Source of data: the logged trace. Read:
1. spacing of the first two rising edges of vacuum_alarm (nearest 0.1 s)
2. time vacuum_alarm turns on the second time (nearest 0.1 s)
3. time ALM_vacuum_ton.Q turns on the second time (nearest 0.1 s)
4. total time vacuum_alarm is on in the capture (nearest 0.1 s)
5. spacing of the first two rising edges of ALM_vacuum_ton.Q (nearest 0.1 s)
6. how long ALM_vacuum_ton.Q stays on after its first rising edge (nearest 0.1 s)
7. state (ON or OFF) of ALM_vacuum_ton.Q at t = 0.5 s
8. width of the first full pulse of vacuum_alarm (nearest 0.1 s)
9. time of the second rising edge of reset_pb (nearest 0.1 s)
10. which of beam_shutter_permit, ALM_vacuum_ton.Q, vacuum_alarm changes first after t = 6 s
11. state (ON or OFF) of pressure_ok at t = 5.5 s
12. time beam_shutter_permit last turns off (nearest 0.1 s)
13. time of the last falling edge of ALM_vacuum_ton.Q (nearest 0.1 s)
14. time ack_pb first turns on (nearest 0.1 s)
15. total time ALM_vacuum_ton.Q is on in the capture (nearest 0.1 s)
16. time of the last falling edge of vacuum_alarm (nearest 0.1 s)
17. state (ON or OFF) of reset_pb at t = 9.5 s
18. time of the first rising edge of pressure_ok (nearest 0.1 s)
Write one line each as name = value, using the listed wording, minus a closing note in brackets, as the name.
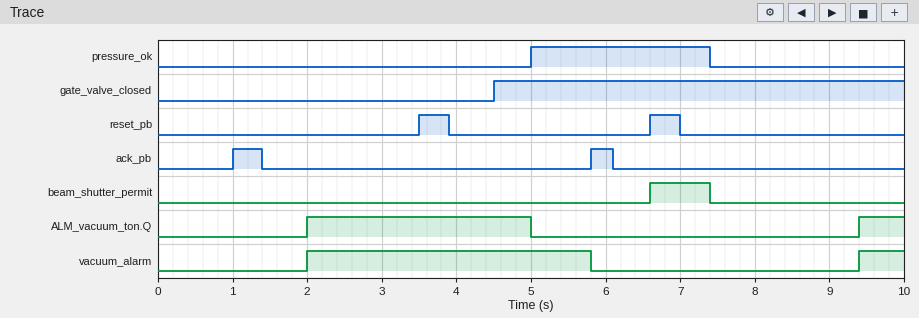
spacing of the first two rising edges of vacuum_alarm = 7.4 s
time vacuum_alarm turns on the second time = 9.4 s
time ALM_vacuum_ton.Q turns on the second time = 9.4 s
total time vacuum_alarm is on in the capture = 4.4 s
spacing of the first two rising edges of ALM_vacuum_ton.Q = 7.4 s
how long ALM_vacuum_ton.Q stays on after its first rising edge = 3.0 s
state (ON or OFF) of ALM_vacuum_ton.Q at t = 0.5 s = OFF
width of the first full pulse of vacuum_alarm = 3.8 s
time of the second rising edge of reset_pb = 6.6 s
which of beam_shutter_permit, ALM_vacuum_ton.Q, vacuum_alarm changes first after t = 6 s = beam_shutter_permit
state (ON or OFF) of pressure_ok at t = 5.5 s = ON
time beam_shutter_permit last turns off = 7.4 s
time of the last falling edge of ALM_vacuum_ton.Q = 5.0 s
time ack_pb first turns on = 1.0 s
total time ALM_vacuum_ton.Q is on in the capture = 3.6 s
time of the last falling edge of vacuum_alarm = 5.8 s
state (ON or OFF) of reset_pb at t = 9.5 s = OFF
time of the first rising edge of pressure_ok = 5.0 s
